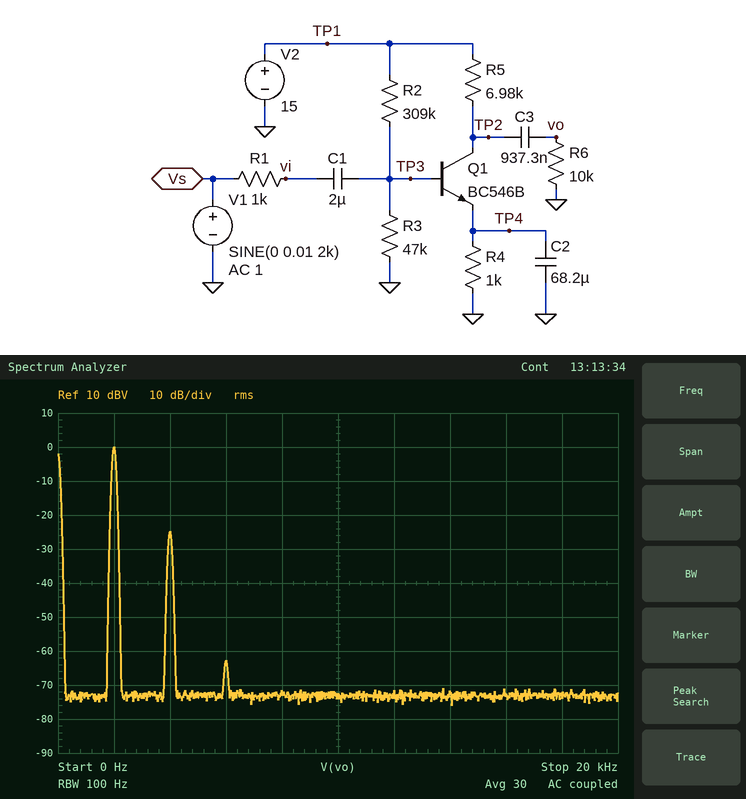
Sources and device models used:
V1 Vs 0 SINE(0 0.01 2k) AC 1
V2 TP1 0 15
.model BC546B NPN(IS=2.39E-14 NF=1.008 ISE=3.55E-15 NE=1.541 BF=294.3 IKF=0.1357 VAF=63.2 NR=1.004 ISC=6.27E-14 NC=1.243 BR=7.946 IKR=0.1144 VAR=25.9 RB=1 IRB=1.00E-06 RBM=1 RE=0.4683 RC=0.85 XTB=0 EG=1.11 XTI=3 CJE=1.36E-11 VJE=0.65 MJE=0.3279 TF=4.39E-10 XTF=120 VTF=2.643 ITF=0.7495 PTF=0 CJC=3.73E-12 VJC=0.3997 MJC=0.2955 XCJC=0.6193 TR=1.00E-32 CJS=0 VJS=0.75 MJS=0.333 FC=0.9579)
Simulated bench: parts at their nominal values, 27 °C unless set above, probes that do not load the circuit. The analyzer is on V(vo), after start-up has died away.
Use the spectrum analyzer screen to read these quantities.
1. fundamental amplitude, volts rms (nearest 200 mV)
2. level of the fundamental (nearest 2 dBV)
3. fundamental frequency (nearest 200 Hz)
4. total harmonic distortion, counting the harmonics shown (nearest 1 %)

1.0 V
0 dBV
2.0 kHz
6 %
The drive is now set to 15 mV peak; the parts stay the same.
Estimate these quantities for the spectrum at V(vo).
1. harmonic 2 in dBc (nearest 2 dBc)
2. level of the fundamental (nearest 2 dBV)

-22 dBc
4 dBV
